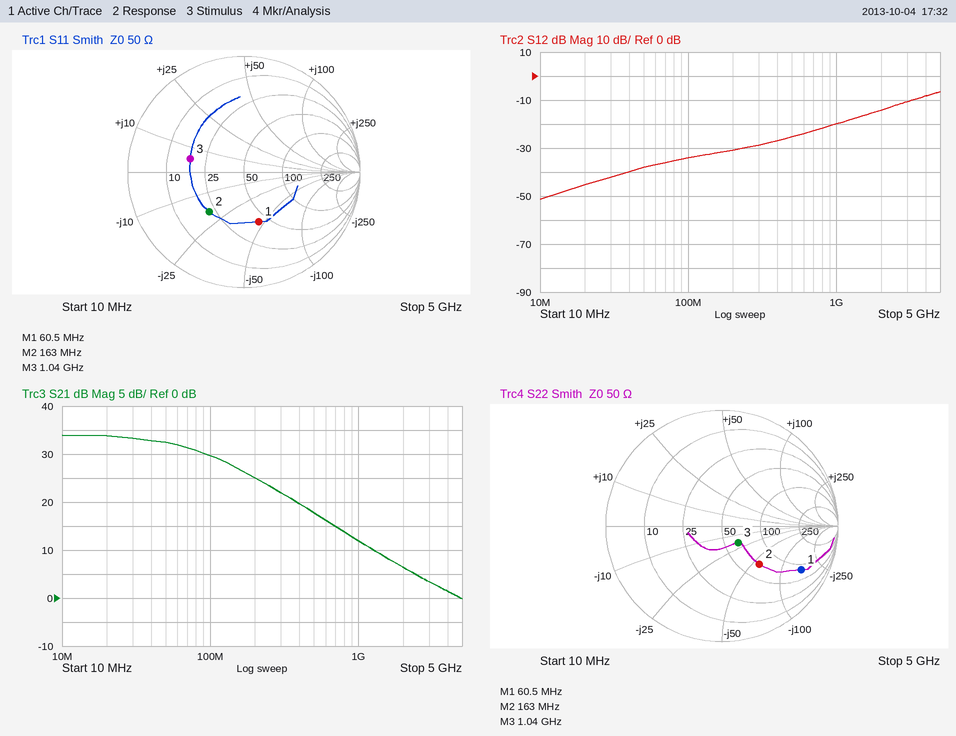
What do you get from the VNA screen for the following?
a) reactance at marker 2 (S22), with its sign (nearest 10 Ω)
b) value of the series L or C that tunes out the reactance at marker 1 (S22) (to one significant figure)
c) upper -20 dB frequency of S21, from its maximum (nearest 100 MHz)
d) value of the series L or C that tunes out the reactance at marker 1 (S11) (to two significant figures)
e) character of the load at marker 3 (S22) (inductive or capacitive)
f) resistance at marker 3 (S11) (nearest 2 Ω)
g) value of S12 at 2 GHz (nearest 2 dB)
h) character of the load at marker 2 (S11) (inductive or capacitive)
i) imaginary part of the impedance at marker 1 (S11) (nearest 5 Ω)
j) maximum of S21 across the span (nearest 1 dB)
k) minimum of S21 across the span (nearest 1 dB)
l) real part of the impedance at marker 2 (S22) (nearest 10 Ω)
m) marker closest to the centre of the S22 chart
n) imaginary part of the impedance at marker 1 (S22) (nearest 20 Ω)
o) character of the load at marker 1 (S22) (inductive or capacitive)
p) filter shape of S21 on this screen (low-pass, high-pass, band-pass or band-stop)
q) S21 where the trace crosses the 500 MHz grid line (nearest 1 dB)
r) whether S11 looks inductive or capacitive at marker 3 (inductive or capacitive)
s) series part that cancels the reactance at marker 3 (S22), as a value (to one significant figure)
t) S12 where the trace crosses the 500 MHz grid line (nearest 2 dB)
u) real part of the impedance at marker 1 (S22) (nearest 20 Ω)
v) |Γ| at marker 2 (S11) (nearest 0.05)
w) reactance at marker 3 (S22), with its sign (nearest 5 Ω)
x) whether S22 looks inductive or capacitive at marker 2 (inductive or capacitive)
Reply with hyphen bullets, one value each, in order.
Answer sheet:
- -60 Ω
- 400 nH
- 800 MHz
- 120 nH
- capacitive
- 18 Ω
- -14 dB
- capacitive
- -45 Ω
- 34 dB
- 0 dB
- 70 Ω
- marker 3
- -160 Ω
- capacitive
- low-pass
- 18 dB
- inductive
- 3 nH
- -26 dB
- 80 Ω
- 0.45
- -20 Ω
- capacitive
